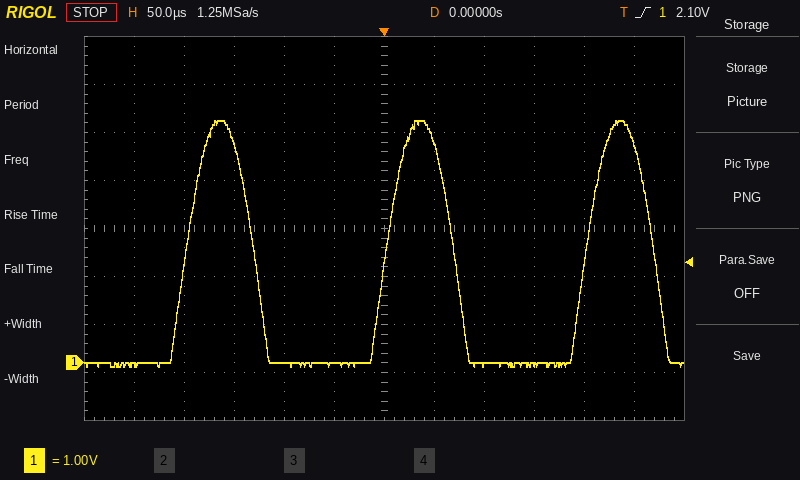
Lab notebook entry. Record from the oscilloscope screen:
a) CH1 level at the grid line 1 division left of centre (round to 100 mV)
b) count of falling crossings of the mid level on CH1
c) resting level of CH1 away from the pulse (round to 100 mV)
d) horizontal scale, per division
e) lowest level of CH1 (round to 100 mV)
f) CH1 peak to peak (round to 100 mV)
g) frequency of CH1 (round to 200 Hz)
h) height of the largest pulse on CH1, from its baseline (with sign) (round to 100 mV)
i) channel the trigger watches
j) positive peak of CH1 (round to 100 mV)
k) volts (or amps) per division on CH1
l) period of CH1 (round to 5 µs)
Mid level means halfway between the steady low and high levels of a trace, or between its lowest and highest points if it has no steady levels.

0.0 V
3
0.0 V
50 µs
-100 mV
5.1 V
5.0 kHz
+5.0 V
CH1
5.0 V
1 V
200 µs
